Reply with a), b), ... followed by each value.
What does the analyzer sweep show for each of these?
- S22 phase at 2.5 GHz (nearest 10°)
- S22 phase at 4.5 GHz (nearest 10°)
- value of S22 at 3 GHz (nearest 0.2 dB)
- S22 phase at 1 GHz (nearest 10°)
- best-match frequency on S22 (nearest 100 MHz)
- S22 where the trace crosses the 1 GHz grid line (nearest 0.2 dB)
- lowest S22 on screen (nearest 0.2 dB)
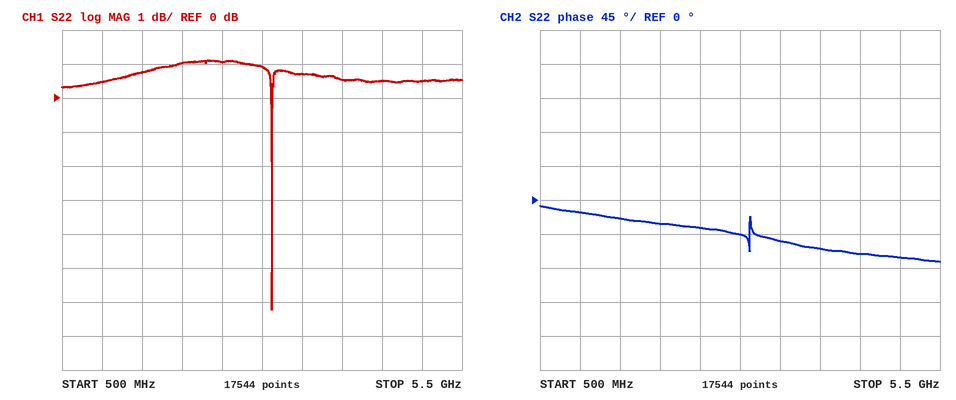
a) -40°
b) -70°
c) 1.0 dB
d) -20°
e) 3.1 GHz
f) 0.4 dB
g) -6.2 dB
